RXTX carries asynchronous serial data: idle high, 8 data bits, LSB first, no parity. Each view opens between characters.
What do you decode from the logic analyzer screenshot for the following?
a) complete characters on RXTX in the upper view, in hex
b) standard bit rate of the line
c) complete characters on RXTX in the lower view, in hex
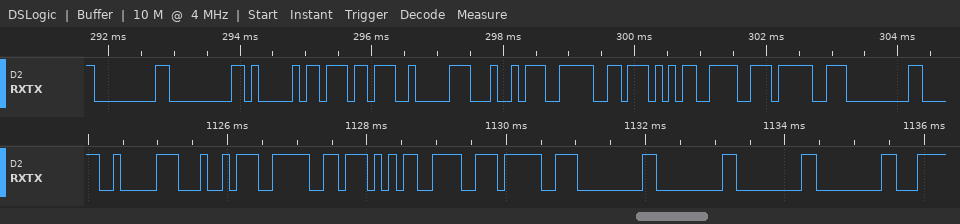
00, 00, 41, B7, 82, A4, 3E, 57, 9E, 9F, 00
9600 baud
82, A4, 3E, 57, 9E, 9F, 00, 00, 00, 00
